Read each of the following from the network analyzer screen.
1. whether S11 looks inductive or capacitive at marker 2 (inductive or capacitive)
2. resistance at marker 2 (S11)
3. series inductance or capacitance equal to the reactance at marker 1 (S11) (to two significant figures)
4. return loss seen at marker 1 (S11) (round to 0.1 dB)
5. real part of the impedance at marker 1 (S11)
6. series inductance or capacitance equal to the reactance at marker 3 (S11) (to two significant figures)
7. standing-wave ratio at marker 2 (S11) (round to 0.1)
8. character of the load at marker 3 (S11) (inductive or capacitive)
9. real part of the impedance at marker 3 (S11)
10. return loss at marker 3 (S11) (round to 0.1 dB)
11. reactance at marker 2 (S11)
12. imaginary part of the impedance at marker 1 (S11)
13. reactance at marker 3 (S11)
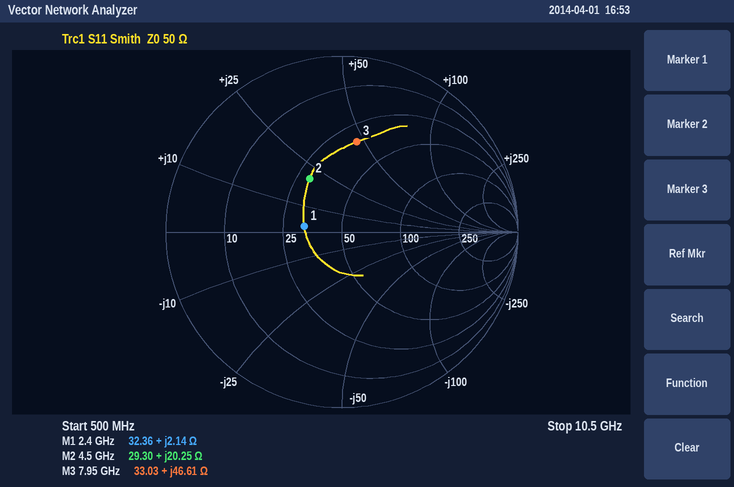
inductive
29.30 Ω
140 pH
13.3 dB
32.36 Ω
930 pH
2.1
inductive
33.03 Ω
5.7 dB
+20.25 Ω
+2.14 Ω
+46.61 Ω
